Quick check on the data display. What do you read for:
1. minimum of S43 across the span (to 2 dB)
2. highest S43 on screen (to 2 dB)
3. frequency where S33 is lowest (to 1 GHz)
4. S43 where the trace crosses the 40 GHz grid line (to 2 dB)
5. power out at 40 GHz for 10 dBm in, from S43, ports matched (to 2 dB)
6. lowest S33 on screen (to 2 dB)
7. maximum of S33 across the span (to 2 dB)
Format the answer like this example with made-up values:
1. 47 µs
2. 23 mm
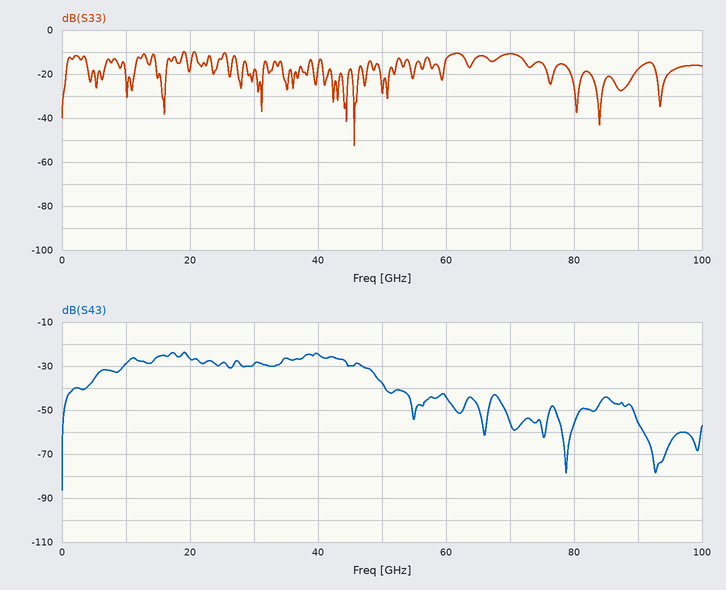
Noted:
1. -86 dB
2. -24 dB
3. 46 GHz
4. -24 dB
5. -14 dBm
6. -52 dB
7. -10 dB
